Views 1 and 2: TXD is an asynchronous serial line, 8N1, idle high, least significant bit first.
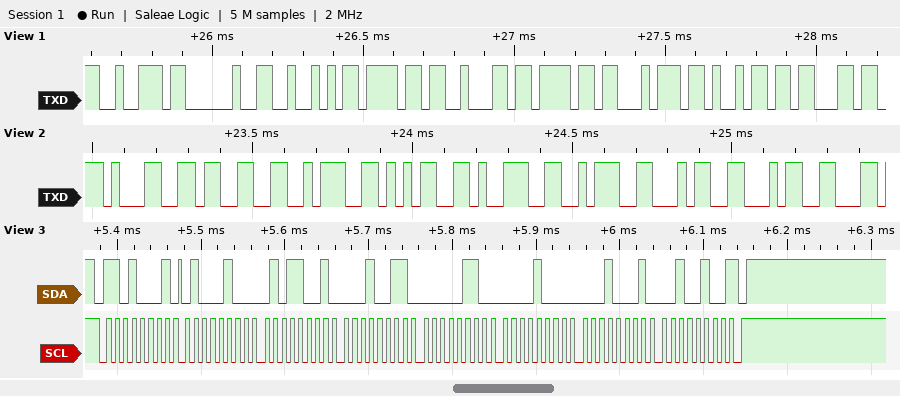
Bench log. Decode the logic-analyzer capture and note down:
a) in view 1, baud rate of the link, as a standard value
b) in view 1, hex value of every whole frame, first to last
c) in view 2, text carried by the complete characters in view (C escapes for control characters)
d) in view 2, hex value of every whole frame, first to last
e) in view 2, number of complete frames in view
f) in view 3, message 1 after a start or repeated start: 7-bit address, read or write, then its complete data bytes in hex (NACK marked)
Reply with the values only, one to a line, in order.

38400 baud
72 20 52 6F 62 6F 74 69 63
"13:59:44"
31 33 3A 35 39 3A 34 34
8
0x68 read: 44 59 13 06 08 11 24 NACK
